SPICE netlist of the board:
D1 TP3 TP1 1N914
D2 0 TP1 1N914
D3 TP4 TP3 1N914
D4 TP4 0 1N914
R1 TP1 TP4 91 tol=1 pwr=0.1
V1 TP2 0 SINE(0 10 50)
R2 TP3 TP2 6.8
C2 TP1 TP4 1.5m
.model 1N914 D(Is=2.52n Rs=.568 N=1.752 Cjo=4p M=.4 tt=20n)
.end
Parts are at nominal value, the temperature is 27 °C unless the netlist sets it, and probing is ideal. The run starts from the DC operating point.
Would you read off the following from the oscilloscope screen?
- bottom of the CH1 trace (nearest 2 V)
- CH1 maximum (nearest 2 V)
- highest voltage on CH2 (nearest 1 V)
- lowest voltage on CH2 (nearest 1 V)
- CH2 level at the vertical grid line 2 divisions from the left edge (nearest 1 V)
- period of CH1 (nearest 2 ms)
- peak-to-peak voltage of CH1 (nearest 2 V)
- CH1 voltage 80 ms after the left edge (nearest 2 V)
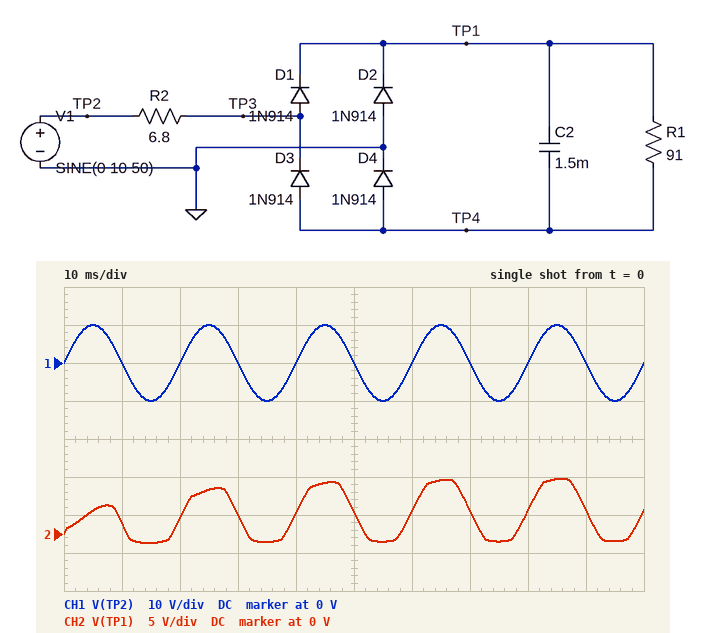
-10 V
10 V
7 V
-1 V
2 V
20 ms
20 V
0 V
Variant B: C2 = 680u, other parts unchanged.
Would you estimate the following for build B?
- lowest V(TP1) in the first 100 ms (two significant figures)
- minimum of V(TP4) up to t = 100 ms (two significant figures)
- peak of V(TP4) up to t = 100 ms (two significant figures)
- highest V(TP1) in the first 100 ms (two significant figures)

-1.1 V
-7.5 V
1.3 V
7.5 V
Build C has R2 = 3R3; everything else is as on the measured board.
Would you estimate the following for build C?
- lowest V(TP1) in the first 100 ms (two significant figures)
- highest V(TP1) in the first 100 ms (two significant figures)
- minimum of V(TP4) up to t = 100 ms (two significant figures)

-1.3 V
8.0 V
-8.0 V
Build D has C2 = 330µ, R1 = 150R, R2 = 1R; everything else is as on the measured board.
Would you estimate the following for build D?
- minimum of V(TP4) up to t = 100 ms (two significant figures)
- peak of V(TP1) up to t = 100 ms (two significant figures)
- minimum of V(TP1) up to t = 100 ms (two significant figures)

-8.9 V
8.9 V
-1.0 V
